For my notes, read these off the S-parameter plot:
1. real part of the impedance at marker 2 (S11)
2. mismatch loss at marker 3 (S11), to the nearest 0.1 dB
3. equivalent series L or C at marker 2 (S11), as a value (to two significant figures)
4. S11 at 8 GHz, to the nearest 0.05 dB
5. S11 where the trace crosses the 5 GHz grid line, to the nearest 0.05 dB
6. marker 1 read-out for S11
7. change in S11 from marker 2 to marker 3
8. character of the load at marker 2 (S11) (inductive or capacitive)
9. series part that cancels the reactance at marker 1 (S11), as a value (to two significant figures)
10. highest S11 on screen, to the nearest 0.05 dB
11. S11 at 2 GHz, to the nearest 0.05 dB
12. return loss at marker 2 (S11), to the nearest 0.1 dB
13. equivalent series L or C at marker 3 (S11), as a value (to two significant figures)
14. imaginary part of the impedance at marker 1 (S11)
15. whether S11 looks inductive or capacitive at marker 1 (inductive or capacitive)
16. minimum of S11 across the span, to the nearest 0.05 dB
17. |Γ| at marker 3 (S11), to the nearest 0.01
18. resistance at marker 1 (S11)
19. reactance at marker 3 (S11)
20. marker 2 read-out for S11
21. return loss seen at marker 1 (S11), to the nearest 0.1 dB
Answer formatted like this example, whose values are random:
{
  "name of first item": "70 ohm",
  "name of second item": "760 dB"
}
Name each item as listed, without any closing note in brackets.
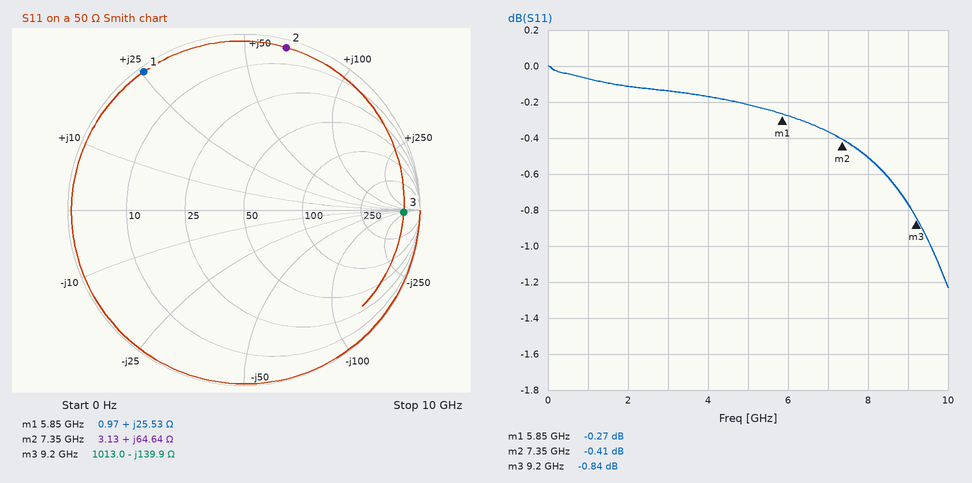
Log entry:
{
  "real part of the impedance at marker 2": "3.13 Ω",
  "mismatch loss at marker 3 (S11), to the nearest 0.1 dB": "7.5 dB",
  "equivalent series L or C at marker 2 (S11), as a value": "1.4 nH",
  "S11 at 8 GHz, to the nearest 0.05 dB": "-0.50 dB",
  "S11 where the trace crosses the 5 GHz grid line, to the nearest 0.05 dB": "-0.20 dB",
  "marker 1 read-out for S11": "-0.27 dB",
  "change in S11 from marker 2 to marker 3": "-0.43 dB",
  "character of the load at marker 2 (S11)": "inductive",
  "series part that cancels the reactance at marker 1 (S11), as a value": "1.1 pF",
  "highest S11 on screen, to the nearest 0.05 dB": "0.00 dB",
  "S11 at 2 GHz, to the nearest 0.05 dB": "-0.10 dB",
  "return loss at marker 2 (S11), to the nearest 0.1 dB": "0.4 dB",
  "equivalent series L or C at marker 3 (S11), as a value": "120 fF",
  "imaginary part of the impedance at marker 1": "+25.53 Ω",
  "whether S11 looks inductive or capacitive at marker 1": "inductive",
  "minimum of S11 across the span, to the nearest 0.05 dB": "-1.25 dB",
  "|Γ| at marker 3 (S11), to the nearest 0.01": "0.91",
  "resistance at marker 1": "0.97 Ω",
  "reactance at marker 3": "-139.9 Ω",
  "marker 2 read-out for S11": "-0.41 dB",
  "return loss seen at marker 1 (S11), to the nearest 0.1 dB": "0.3 dB"
}
